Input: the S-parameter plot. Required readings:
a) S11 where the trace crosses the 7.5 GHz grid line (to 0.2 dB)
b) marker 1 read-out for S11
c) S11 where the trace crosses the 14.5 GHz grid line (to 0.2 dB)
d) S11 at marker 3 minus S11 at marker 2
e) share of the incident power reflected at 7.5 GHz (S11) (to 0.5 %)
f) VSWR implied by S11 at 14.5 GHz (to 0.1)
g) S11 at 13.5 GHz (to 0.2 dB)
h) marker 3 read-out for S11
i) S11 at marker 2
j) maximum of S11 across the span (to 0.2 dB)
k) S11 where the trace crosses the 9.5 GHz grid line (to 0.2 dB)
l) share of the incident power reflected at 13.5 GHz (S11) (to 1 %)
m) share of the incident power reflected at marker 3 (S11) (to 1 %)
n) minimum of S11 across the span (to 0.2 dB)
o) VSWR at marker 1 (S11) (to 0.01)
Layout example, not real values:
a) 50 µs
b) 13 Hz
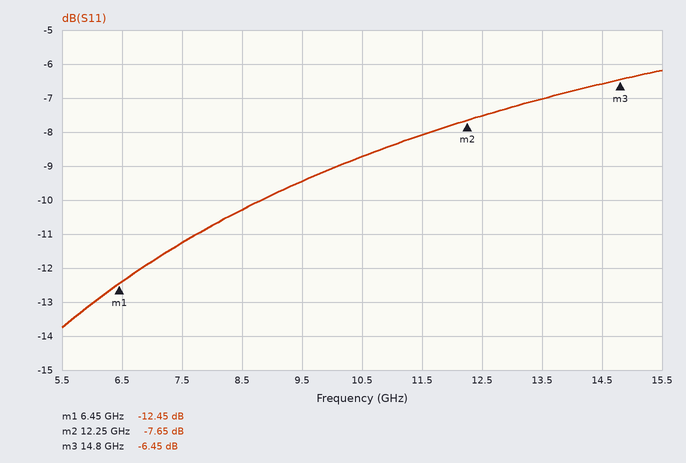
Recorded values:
a) -11.2 dB
b) -12.45 dB
c) -6.6 dB
d) 1.20 dB
e) 7.5 %
f) 2.8
g) -7.0 dB
h) -6.45 dB
i) -7.65 dB
j) -6.2 dB
k) -9.4 dB
l) 20 %
m) 23 %
n) -13.8 dB
o) 1.63
